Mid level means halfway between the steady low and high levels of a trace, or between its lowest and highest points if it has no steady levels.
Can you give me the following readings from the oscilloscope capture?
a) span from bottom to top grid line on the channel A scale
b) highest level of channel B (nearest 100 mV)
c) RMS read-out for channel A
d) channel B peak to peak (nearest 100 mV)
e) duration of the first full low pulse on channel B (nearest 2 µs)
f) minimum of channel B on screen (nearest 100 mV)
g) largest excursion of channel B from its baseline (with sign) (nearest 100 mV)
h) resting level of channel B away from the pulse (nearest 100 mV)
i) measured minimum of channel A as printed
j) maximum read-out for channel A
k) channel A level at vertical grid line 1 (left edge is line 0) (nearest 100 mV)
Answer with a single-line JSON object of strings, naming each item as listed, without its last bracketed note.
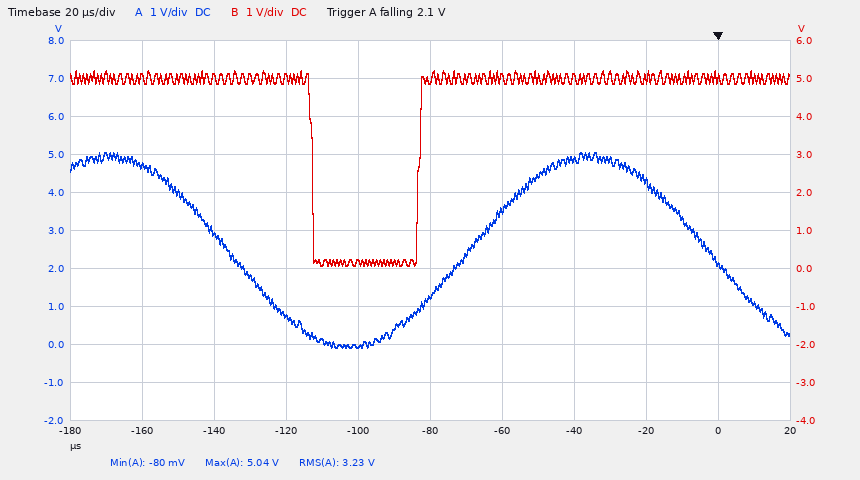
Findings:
{"span from bottom to top grid line on the channel A scale": "10 V", "highest level of channel B": "5.2 V", "RMS read-out for channel A": "3.23 V", "channel B peak to peak": "5.1 V", "duration of the first full low pulse on channel B": "30 µs", "minimum of channel B on screen": "100 mV", "largest excursion of channel B from its baseline (with sign)": "-4.9 V", "resting level of channel B away from the pulse": "5.0 V", "measured minimum of channel A as printed": "-80 mV", "maximum read-out for channel A": "5.04 V", "channel A level at vertical grid line 1 (left edge is line 0)": "4.7 V"}
